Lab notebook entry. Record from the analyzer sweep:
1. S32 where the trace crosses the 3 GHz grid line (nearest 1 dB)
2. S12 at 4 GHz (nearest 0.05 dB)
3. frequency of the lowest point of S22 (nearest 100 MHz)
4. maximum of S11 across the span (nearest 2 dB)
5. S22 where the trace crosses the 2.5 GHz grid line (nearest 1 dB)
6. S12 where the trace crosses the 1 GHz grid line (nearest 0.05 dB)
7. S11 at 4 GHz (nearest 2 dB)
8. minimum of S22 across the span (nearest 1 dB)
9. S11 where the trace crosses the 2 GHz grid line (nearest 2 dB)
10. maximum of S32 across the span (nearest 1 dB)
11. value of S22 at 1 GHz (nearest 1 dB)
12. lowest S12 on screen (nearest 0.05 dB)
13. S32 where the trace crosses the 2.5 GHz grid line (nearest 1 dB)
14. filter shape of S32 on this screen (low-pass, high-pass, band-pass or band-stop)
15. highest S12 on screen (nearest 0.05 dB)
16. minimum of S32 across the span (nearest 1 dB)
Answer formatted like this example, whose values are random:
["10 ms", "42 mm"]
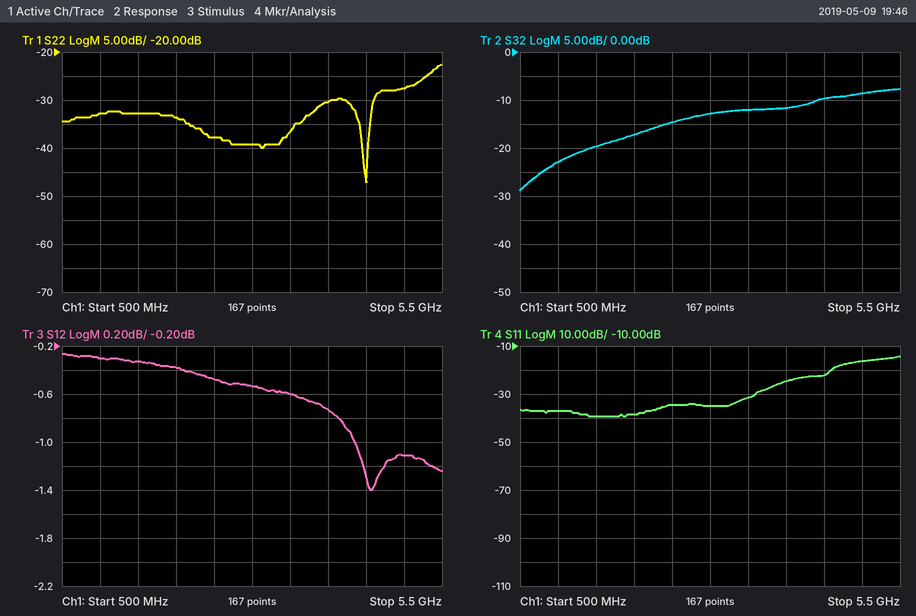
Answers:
["-13 dB", "-0.75 dB", "4.5 GHz", "-14 dB", "-38 dB", "-0.30 dB", "-24 dB", "-47 dB", "-38 dB", "-8 dB", "-33 dB", "-1.40 dB", "-15 dB", "high-pass", "-0.25 dB", "-29 dB"]
